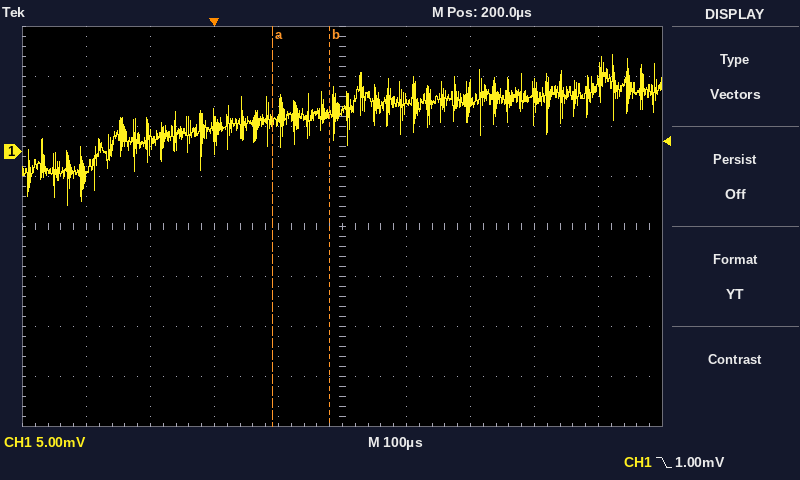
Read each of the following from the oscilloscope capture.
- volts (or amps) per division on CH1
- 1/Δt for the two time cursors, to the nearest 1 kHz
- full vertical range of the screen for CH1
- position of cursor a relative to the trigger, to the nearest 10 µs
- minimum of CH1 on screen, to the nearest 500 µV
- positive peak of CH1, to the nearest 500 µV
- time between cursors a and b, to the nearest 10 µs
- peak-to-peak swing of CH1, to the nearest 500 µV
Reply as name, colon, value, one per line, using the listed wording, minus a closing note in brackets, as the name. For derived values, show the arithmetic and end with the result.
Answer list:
volts (or amps) per division on CH1: 5 mV
1/Δt for the two time cursors, to the nearest 1 kHz: 1 / 90 µs ≈ 11 kHz
full vertical range of the screen for CH1: 40 mV
position of cursor a relative to the trigger, to the nearest 10 µs: +90 µs
minimum of CH1 on screen, to the nearest 500 µV: -5.5 mV
positive peak of CH1, to the nearest 500 µV: 9.5 mV
time between cursors a and b, to the nearest 10 µs: 90 µs
peak-to-peak swing of CH1, to the nearest 500 µV: 9.5 mV − (-5.5 mV) = 15.0 mV
